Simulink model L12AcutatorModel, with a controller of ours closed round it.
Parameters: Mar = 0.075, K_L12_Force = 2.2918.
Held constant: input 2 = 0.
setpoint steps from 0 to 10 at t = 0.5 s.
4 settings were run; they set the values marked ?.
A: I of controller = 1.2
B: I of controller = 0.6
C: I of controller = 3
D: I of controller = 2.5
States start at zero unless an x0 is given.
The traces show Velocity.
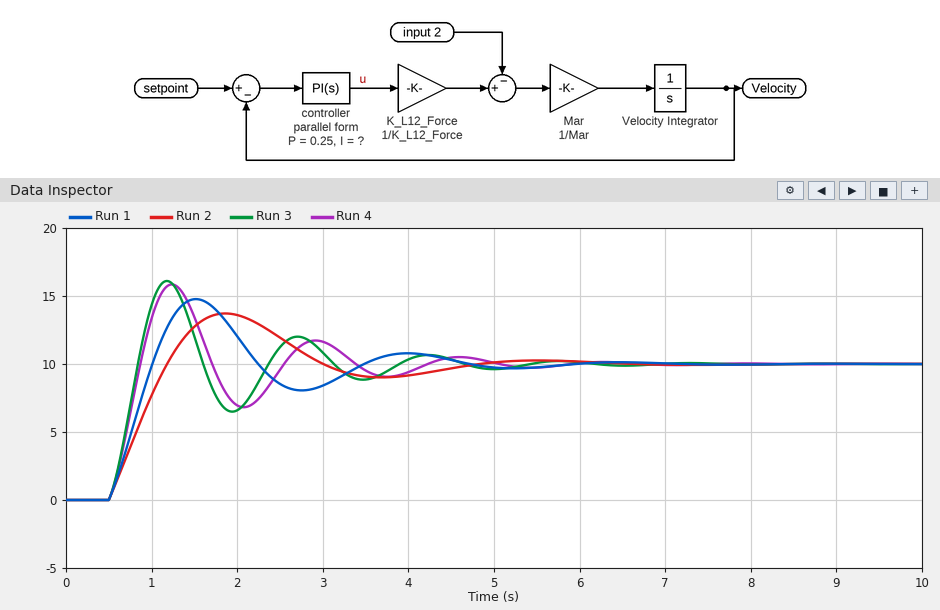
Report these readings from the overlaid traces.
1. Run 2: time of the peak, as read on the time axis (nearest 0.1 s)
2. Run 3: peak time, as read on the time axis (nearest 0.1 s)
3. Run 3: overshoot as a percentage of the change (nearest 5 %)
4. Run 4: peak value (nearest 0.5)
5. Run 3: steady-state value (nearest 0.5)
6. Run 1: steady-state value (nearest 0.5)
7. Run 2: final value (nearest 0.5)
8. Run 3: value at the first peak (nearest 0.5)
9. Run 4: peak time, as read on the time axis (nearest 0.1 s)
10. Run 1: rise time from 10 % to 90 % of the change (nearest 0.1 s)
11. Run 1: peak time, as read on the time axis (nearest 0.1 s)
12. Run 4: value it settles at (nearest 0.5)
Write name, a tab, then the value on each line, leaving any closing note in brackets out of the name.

Run 2: time of the peak, as read on the time axis	1.9 s
Run 3: peak time, as read on the time axis	1.2 s
Run 3: overshoot as a percentage of the change	60 %
Run 4: peak value	16.0
Run 3: steady-state value	10.0
Run 1: steady-state value	10.0
Run 2: final value	10.0
Run 3: value at the first peak	16.0
Run 4: peak time, as read on the time axis	1.2 s
Run 1: rise time from 10 % to 90 % of the change	0.4 s
Run 1: peak time, as read on the time axis	1.5 s
Run 4: value it settles at	10.0
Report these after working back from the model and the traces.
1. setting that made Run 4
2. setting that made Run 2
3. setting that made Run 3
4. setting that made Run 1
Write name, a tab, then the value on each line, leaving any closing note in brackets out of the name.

setting that made Run 4	D
setting that made Run 2	B
setting that made Run 3	C
setting that made Run 1	A
